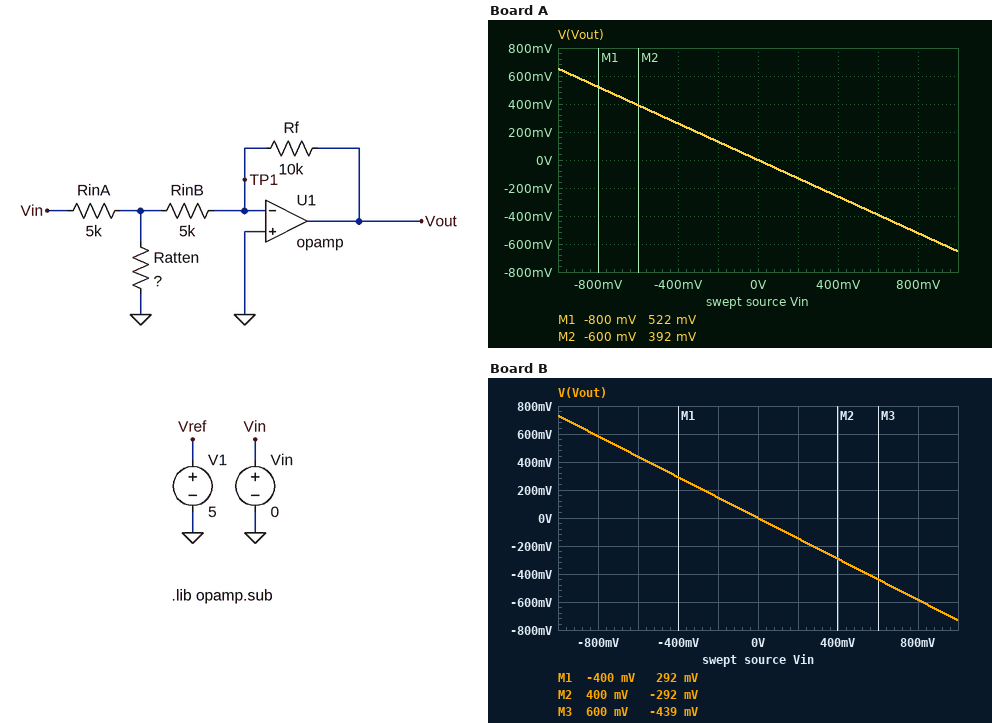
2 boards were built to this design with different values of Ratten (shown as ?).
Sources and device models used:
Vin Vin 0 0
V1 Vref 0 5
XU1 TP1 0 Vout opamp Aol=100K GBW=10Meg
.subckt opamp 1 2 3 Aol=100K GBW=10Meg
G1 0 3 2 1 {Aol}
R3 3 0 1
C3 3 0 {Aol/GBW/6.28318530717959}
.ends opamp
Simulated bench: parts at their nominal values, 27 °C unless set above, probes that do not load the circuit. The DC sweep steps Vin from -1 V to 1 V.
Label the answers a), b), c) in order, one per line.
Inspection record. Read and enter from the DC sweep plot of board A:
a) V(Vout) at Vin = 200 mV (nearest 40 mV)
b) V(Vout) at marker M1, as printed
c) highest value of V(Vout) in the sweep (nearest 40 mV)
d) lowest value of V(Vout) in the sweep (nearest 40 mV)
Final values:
a) -120 mV
b) 522 mV
c) 640 mV
d) -640 mV
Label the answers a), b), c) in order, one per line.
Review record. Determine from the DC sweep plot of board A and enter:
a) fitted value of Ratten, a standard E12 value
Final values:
a) 4.7 kΩ
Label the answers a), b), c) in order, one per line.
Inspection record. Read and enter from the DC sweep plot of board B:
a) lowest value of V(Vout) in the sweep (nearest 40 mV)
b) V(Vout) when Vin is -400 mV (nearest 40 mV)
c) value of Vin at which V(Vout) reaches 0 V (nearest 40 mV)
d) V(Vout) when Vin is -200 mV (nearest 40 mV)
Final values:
a) -720 mV
b) 280 mV
c) 0 V
d) 160 mV
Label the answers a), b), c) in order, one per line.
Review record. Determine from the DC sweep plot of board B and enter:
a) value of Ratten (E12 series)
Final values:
a) 6.8 kΩ
